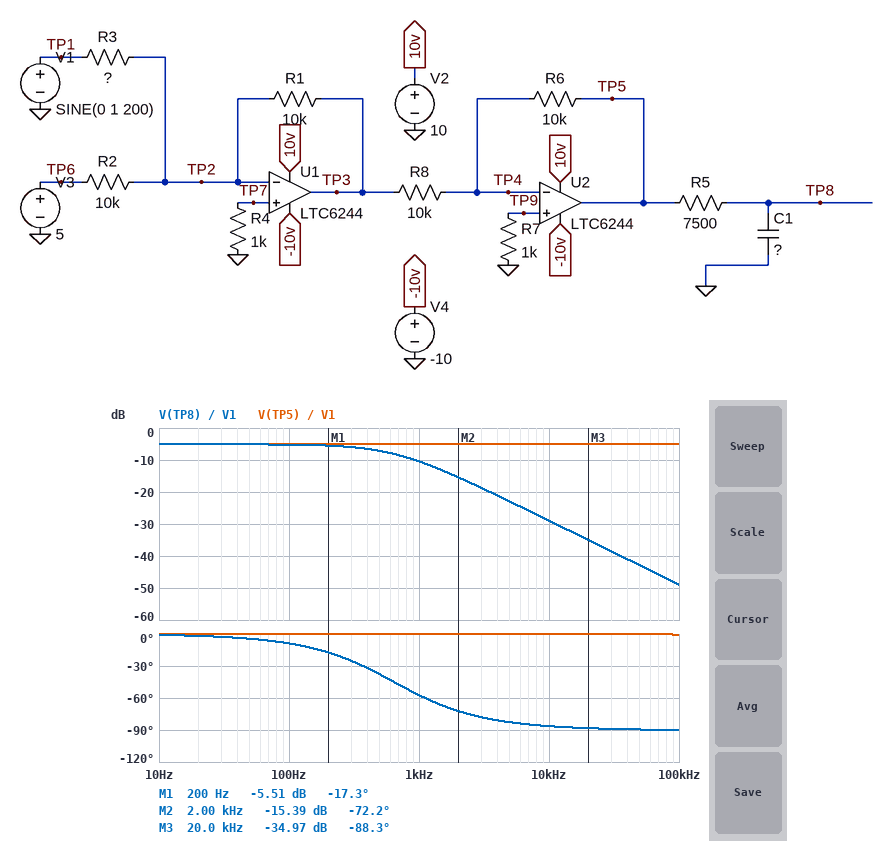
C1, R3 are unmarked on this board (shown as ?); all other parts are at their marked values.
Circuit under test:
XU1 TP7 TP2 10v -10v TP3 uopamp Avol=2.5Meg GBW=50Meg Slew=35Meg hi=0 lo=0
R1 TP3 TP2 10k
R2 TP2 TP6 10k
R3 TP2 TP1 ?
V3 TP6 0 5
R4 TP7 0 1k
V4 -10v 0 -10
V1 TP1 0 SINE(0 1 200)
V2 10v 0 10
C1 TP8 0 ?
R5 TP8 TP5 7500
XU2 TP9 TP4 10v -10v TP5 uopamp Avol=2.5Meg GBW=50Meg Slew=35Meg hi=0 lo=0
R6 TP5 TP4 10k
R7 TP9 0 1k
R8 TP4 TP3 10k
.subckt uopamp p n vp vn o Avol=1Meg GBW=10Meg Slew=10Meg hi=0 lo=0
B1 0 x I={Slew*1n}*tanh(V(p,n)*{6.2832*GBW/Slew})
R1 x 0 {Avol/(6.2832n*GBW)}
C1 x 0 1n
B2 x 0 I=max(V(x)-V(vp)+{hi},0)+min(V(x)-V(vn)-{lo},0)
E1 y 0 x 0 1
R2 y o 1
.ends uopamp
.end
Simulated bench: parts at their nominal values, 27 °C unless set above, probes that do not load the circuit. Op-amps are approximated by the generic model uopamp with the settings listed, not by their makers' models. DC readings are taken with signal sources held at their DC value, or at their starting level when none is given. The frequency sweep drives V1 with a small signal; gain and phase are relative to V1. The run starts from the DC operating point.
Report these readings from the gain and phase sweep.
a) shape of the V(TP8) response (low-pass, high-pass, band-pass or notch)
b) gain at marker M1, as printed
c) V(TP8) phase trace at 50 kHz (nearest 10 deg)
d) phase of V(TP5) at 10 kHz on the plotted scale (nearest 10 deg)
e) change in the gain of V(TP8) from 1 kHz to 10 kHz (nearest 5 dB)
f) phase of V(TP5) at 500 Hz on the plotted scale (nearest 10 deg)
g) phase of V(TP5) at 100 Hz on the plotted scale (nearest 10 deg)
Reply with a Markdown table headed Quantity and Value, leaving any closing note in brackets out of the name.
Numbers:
| Quantity | Value |
|---|---|
| shape of the V(TP8) response | low-pass |
| gain at marker M1, as printed | -5.51 dB |
| V(TP8) phase trace at 50 kHz | -90 deg |
| phase of V(TP5) at 10 kHz on the plotted scale | 0 deg |
| change in the gain of V(TP8) from 1 kHz to 10 kHz | -20 dB |
| phase of V(TP5) at 500 Hz on the plotted scale | 0 deg |
| phase of V(TP5) at 100 Hz on the plotted scale | 0 deg |
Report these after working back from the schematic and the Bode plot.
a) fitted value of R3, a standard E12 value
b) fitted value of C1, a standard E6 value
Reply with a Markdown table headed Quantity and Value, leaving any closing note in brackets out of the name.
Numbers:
| Quantity | Value |
|---|---|
| fitted value of R3, a standard E12 value | 18 kΩ |
| fitted value of C1, a standard E6 value | 33 nF |
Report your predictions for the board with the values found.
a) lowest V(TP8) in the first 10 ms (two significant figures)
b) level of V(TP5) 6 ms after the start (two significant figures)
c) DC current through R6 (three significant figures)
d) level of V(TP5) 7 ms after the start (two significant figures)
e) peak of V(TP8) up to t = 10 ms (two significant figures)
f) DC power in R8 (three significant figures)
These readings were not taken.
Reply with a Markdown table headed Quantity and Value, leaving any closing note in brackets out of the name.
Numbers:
| Quantity | Value |
|---|---|
| lowest V(TP8) in the first 10 ms | 4.5 V |
| level of V(TP5) 6 ms after the start | 5.5 V |
| DC current through R6 | 500 µA |
| level of V(TP5) 7 ms after the start | 5.3 V |
| peak of V(TP8) up to t = 10 ms | 5.5 V |
| DC power in R8 | 2.50 mW |
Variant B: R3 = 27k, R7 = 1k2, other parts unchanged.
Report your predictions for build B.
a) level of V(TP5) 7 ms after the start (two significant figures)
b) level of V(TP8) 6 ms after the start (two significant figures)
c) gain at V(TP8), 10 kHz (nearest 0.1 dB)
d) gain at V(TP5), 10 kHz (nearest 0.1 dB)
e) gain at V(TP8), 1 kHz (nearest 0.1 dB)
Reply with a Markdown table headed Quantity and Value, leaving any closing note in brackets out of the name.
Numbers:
| Quantity | Value |
|---|---|
| level of V(TP5) 7 ms after the start | 5.2 V |
| level of V(TP8) 6 ms after the start | 5.3 V |
| gain at V(TP8), 10 kHz | -32.5 dB |
| gain at V(TP5), 10 kHz | -8.6 dB |
| gain at V(TP8), 1 kHz | -14.0 dB |
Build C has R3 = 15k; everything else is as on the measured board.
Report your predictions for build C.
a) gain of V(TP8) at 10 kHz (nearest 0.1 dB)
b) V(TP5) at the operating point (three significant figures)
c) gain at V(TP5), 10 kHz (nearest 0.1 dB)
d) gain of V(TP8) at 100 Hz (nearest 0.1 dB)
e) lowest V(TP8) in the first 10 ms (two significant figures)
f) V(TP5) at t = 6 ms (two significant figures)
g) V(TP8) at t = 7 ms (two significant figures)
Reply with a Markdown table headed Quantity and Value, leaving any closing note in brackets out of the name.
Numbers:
| Quantity | Value |
|---|---|
| gain of V(TP8) at 10 kHz | -27.4 dB |
| V(TP5) at the operating point | 5.00 V |
| gain at V(TP5), 10 kHz | -3.5 dB |
| gain of V(TP8) at 100 Hz | -3.6 dB |
| lowest V(TP8) in the first 10 ms | 4.4 V |
| V(TP5) at t = 6 ms | 5.6 V |
| V(TP8) at t = 7 ms | 5.5 V |
